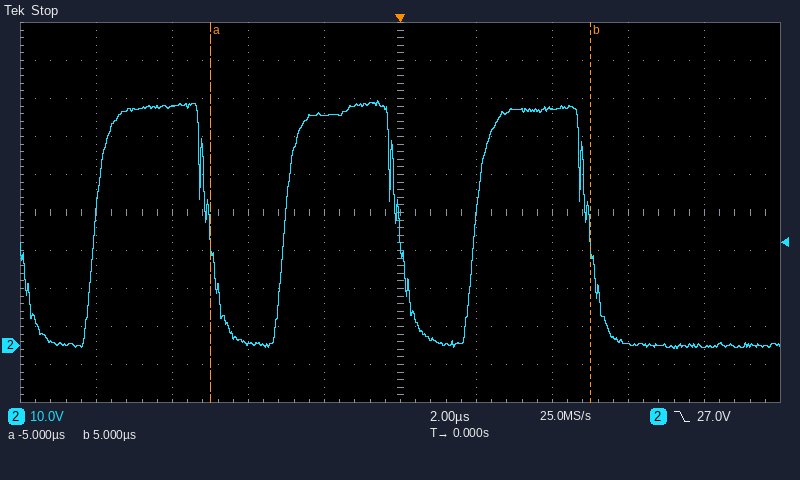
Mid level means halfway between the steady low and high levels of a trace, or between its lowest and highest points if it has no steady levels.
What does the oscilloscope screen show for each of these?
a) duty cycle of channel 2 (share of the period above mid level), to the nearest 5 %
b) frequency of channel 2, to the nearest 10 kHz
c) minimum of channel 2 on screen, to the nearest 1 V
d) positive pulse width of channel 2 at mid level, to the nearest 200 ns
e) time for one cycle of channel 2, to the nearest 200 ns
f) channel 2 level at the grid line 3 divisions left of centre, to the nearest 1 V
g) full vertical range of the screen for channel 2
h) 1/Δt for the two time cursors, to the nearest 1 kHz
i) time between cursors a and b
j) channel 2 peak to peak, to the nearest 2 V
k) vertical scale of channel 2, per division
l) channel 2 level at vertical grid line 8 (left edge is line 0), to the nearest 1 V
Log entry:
60 %
200 kHz
-1 V
3.0 µs
5.0 µs
63 V
100 V
100 kHz
10.0 µs
66 V
10 V
0 V
